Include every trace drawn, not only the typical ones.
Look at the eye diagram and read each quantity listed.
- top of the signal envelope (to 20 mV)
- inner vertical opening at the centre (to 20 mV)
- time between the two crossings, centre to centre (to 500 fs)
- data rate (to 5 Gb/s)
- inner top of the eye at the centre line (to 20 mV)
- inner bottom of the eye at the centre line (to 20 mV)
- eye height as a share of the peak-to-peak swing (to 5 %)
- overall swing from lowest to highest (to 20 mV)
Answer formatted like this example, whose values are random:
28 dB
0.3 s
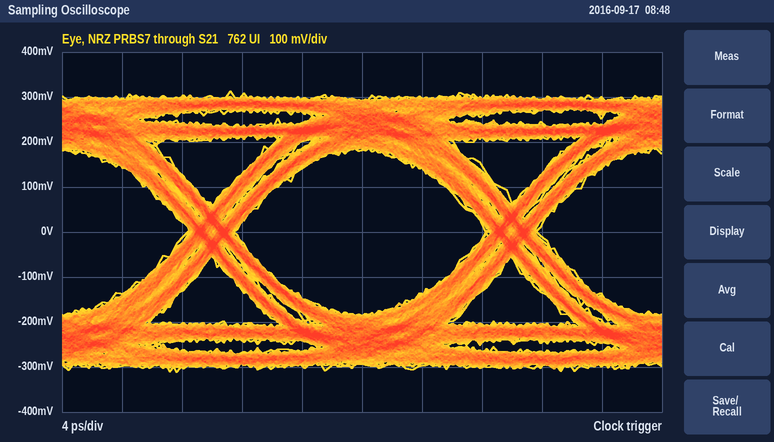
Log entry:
320 mV
360 mV
20.0 ps
50 Gb/s
180 mV
-180 mV
60 %
620 mV
